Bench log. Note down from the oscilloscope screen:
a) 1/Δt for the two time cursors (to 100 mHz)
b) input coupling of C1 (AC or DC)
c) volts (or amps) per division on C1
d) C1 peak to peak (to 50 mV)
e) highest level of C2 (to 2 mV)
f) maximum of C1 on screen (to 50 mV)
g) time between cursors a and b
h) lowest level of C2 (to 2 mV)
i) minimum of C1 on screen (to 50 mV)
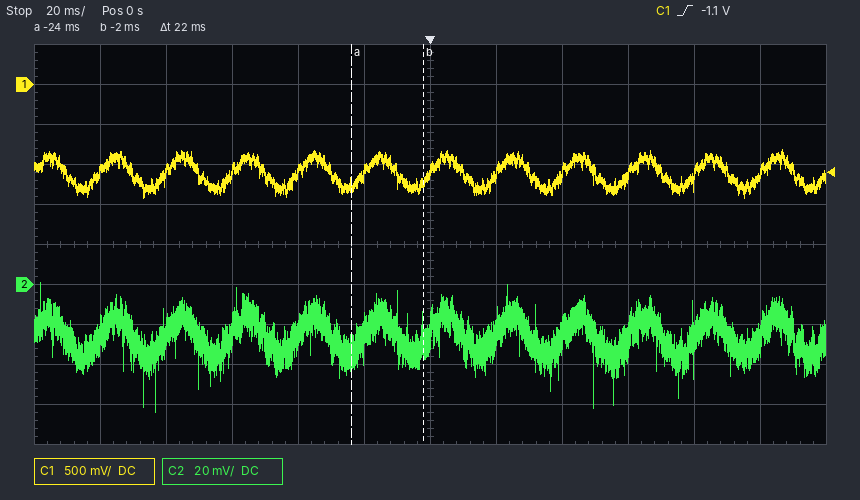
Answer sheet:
45.5 Hz
DC
500 mV
600 mV
2 mV
-800 mV
22 ms
-64 mV
-1.40 V
